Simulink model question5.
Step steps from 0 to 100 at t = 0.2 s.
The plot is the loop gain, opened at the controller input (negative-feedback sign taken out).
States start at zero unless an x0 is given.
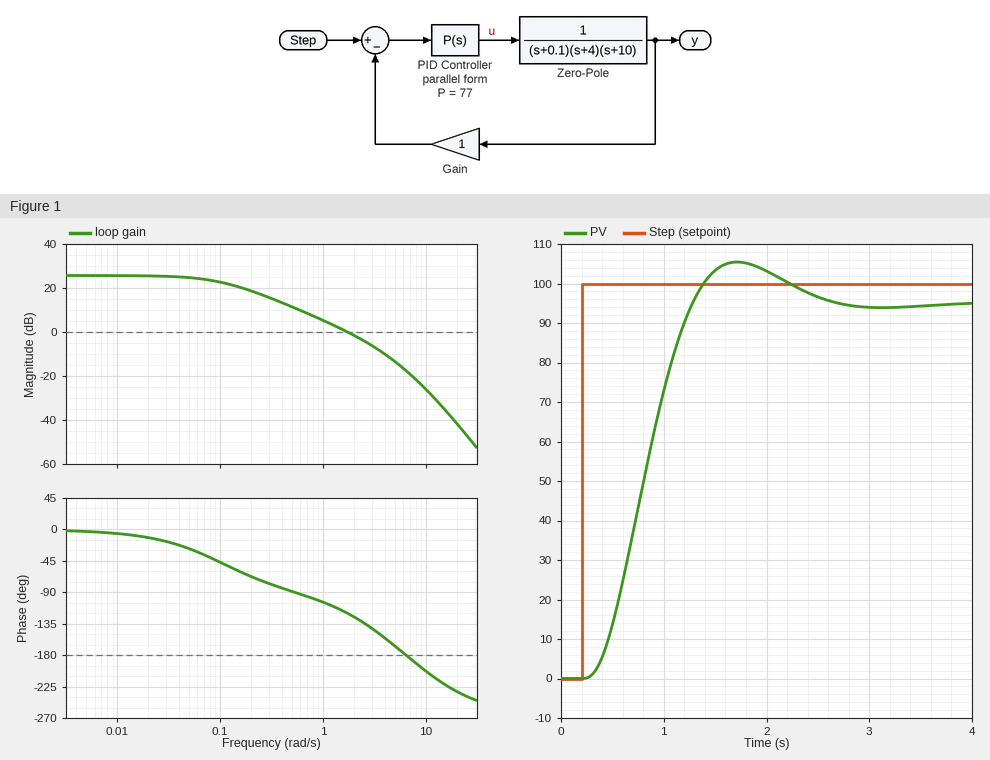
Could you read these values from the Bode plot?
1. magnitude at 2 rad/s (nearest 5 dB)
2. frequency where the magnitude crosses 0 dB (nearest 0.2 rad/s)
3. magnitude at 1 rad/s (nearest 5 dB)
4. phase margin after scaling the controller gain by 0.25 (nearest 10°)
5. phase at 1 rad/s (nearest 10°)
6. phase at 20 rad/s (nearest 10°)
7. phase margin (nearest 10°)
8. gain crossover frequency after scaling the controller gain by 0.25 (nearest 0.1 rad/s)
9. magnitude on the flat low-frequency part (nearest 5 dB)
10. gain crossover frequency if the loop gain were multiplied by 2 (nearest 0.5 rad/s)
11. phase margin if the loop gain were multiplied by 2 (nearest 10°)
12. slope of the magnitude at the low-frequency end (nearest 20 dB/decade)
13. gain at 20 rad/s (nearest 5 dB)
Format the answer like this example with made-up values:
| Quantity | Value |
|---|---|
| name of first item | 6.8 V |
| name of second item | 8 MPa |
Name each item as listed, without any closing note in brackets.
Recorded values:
| Quantity | Value |
|---|---|
| magnitude at 2 rad/s | 0 dB |
| frequency where the magnitude crosses 0 dB | 1.8 rad/s |
| magnitude at 1 rad/s | 5 dB |
| phase margin after scaling the controller gain by 0.25 | 90° |
| phase at 1 rad/s | -100° |
| phase at 20 rad/s | -230° |
| phase margin | 60° |
| gain crossover frequency after scaling the controller gain by 0.25 | 0.5 rad/s |
| magnitude on the flat low-frequency part | 25 dB |
| gain crossover frequency if the loop gain were multiplied by 2 | 3.0 rad/s |
| phase margin if the loop gain were multiplied by 2 | 40° |
| slope of the magnitude at the low-frequency end | 0 dB/decade |
| gain at 20 rad/s | -40 dB |
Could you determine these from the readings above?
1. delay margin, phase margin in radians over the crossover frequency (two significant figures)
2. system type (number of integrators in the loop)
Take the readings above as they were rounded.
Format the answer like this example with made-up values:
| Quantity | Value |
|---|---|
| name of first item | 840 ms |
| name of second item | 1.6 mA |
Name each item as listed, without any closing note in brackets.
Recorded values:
| Quantity | Value |
|---|---|
| delay margin, phase margin in radians over the crossover frequency | 0.58 s |
| system type | 0 |
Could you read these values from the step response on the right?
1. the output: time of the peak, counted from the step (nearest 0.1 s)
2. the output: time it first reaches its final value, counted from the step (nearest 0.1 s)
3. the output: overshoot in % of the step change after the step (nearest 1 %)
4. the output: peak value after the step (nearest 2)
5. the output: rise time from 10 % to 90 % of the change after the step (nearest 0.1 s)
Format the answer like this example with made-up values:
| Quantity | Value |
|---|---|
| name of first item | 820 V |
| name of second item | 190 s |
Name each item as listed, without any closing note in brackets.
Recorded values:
| Quantity | Value |
|---|---|
| the output: time of the peak, counted from the step | 1.5 s |
| the output: time it first reaches its final value, counted from the step | 1.1 s |
| the output: overshoot in % of the step change after the step | 11 % |
| the output: peak value after the step | 106 |
| the output: rise time from 10 % to 90 % of the change after the step | 0.7 s |
